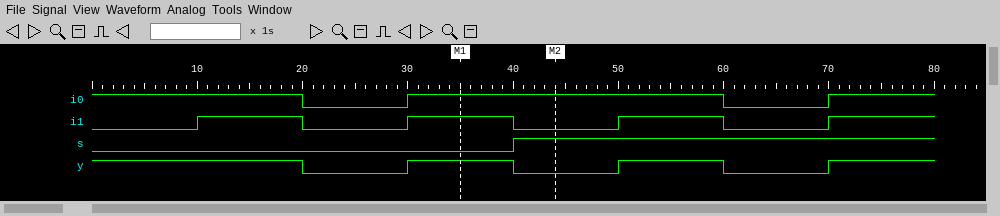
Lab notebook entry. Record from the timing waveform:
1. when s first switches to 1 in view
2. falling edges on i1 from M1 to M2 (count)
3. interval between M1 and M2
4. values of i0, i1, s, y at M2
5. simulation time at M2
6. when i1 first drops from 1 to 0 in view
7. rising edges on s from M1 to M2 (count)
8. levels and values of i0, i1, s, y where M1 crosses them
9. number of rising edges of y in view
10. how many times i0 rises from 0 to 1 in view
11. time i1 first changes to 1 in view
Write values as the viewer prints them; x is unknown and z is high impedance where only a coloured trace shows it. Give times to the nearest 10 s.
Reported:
40 s
1
10 s
i0=1, i1=0, s=1, y=0
40 s
20 s
1
i0=1, i1=1, s=0, y=1
3
2
10 s
